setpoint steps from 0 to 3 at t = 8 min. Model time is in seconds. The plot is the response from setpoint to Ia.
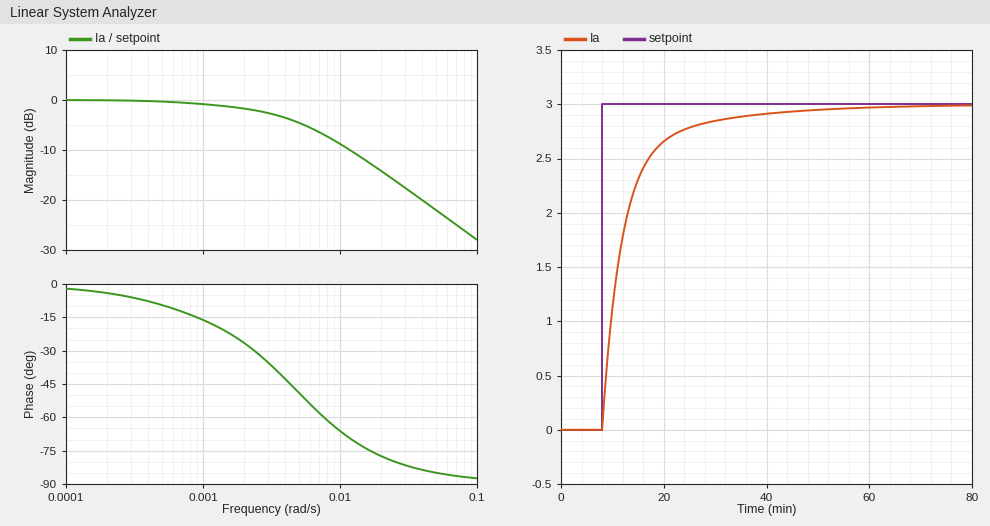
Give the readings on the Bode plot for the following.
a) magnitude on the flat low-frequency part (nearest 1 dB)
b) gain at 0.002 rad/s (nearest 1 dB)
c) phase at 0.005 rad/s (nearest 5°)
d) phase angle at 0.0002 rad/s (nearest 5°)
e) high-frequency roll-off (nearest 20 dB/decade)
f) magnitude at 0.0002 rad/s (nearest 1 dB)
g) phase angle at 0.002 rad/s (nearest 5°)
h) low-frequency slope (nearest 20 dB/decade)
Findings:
0 dB
-2 dB
-50°
-5°
-20 dB/decade
0 dB
-25°
0 dB/decade
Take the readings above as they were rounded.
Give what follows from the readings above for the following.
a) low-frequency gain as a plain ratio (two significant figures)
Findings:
1.0
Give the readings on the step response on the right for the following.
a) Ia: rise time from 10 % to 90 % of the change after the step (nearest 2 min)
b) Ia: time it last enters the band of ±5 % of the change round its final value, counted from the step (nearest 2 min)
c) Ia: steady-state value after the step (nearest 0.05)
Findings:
12 min
22 min
3.00
